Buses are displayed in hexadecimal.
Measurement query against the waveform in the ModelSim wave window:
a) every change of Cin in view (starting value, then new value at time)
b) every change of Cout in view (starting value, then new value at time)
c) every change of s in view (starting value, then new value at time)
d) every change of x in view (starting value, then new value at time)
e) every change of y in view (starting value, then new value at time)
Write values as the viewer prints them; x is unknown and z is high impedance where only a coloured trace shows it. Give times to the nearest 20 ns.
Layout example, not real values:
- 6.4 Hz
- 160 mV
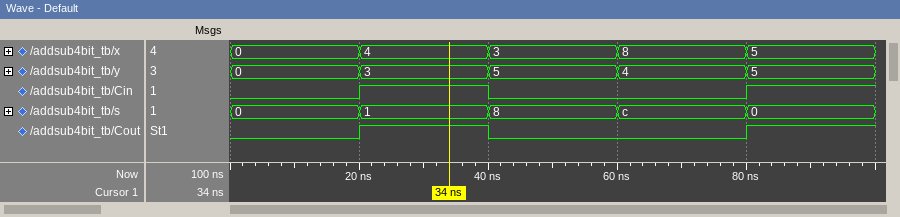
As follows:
- 0, 1 at 20 ns, 0 at 40 ns, 1 at 80 ns
- 0, 1 at 20 ns, 0 at 40 ns, 1 at 80 ns
- 0, 1 at 20 ns, 8 at 40 ns, c at 60 ns, 0 at 80 ns
- 0, 4 at 20 ns, 3 at 40 ns, 8 at 60 ns, 5 at 80 ns
- 0, 3 at 20 ns, 5 at 40 ns, 4 at 60 ns, 5 at 80 ns
